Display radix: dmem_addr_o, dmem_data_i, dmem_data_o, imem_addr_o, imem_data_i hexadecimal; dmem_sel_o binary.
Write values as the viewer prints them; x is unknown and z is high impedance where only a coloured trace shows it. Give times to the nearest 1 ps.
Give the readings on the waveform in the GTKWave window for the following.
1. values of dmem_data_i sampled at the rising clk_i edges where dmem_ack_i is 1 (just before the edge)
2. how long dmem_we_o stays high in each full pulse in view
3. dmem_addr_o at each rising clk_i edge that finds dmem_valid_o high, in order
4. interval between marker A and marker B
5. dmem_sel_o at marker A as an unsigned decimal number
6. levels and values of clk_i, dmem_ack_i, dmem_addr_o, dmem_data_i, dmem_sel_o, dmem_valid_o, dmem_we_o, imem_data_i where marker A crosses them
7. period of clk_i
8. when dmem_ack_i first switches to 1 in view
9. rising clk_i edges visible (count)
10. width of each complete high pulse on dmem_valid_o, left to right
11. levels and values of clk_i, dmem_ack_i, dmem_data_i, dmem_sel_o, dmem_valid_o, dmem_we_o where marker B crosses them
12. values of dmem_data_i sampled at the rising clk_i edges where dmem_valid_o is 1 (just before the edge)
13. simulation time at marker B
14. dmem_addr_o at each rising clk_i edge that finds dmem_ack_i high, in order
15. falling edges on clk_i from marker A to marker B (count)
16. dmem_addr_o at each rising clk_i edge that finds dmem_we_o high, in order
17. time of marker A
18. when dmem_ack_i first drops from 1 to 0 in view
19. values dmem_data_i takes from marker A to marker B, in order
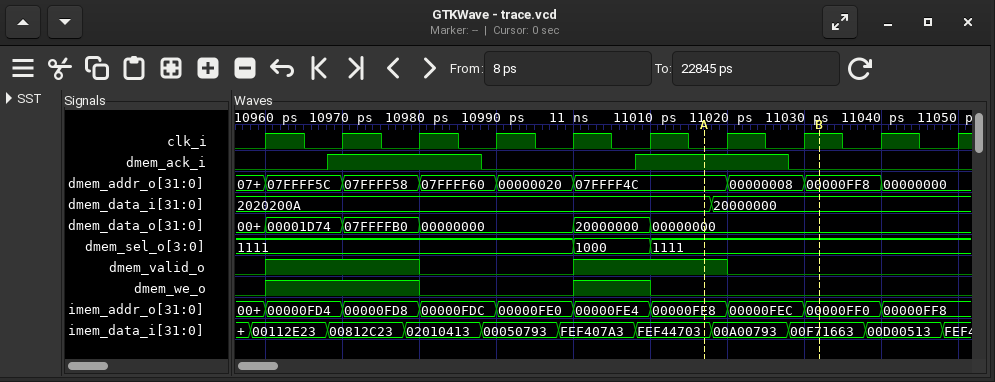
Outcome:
2020200A, 2020200A, 2020200A, 20000000
20 ps, 10 ps
07FFFF5C, 07FFFF58, 07FFFF4C, 07FFFF4C
15 ps
15
clk_i=0, dmem_ack_i=1, dmem_addr_o=07FFFF4C, dmem_data_i=2020200A, dmem_sel_o=1111, dmem_valid_o=1, dmem_we_o=0, imem_data_i=FEF44703
10 ps
10968 ps
10
20 ps, 20 ps
clk_i=1, dmem_ack_i=0, dmem_data_i=20000000, dmem_sel_o=1111, dmem_valid_o=0, dmem_we_o=0
2020200A, 2020200A, 2020200A, 20000000
11032 ps
07FFFF5C, 07FFFF58, 07FFFF4C, 07FFFF4C
1
07FFFF5C, 07FFFF58, 07FFFF4C
11017 ps
10988 ps
2020200A, 20000000
